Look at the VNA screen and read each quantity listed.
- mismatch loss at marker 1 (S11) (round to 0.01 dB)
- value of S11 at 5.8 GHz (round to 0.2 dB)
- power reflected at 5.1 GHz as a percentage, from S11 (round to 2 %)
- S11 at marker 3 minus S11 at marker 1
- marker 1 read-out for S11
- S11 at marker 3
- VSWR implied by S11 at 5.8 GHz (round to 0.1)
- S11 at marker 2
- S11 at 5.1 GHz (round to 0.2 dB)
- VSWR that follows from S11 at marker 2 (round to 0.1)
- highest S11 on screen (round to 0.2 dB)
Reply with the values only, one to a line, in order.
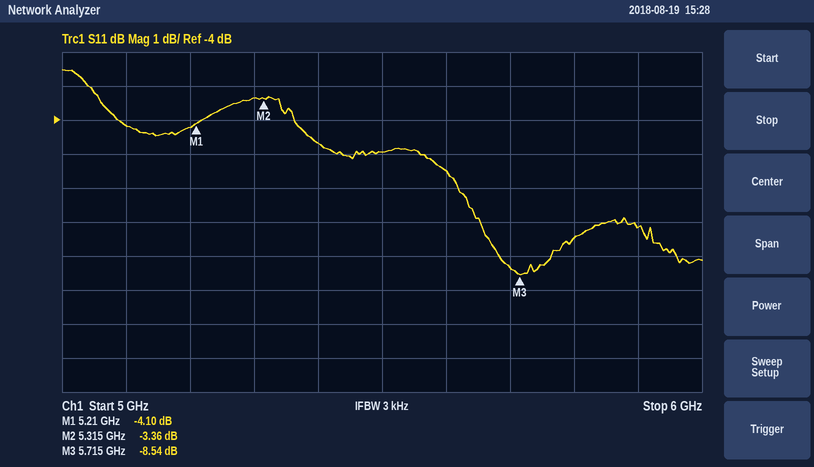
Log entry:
2.14 dB
-7.4 dB
38 %
-4.44 dB
-4.10 dB
-8.54 dB
2.5
-3.36 dB
-4.2 dB
5.2
-2.6 dB
